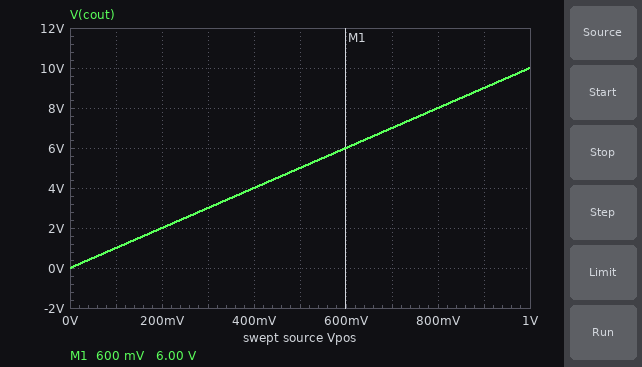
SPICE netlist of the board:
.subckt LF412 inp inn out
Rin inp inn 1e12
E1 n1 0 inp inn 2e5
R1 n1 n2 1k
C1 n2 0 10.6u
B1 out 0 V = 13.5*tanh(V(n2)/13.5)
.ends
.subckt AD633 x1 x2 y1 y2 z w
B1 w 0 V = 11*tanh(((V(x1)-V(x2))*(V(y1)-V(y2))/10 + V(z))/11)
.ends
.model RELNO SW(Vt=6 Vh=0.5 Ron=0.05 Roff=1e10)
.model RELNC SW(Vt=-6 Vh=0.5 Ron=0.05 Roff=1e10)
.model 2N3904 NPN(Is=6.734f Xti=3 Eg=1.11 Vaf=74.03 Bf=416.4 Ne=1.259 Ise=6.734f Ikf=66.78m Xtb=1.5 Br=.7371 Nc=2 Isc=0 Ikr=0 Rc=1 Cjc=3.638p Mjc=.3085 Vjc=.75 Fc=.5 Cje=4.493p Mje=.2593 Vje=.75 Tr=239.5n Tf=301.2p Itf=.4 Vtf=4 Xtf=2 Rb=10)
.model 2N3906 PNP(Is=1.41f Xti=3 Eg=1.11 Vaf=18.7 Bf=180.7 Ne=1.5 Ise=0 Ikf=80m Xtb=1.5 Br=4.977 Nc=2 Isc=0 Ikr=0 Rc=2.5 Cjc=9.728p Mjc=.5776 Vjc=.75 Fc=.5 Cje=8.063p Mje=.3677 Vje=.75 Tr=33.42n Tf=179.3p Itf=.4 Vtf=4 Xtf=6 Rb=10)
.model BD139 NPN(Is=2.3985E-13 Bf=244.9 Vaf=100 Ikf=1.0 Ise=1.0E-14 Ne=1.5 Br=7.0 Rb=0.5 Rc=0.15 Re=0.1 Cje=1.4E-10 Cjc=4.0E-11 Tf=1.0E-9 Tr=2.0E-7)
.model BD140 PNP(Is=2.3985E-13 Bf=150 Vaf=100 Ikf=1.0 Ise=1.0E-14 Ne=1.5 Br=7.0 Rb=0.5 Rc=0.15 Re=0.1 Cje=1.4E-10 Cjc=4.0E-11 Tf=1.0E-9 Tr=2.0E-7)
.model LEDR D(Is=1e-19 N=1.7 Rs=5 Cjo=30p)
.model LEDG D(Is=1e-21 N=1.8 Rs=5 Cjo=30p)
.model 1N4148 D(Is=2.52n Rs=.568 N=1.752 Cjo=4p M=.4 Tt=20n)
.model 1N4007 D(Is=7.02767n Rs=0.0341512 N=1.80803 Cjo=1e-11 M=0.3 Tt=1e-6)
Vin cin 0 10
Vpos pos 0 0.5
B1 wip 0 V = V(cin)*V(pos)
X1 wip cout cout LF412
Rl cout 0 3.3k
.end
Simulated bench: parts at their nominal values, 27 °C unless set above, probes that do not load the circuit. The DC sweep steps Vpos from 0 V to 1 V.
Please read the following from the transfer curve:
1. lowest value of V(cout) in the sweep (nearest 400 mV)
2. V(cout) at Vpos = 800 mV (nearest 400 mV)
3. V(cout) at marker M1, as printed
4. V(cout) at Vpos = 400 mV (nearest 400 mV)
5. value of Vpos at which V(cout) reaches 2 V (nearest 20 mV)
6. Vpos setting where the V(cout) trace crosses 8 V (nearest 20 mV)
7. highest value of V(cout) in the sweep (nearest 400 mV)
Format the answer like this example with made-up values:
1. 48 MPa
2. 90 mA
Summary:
1. 0 V
2. 8.0 V
3. 6.00 V
4. 4.0 V
5. 200 mV
6. 800 mV
7. 10.0 V
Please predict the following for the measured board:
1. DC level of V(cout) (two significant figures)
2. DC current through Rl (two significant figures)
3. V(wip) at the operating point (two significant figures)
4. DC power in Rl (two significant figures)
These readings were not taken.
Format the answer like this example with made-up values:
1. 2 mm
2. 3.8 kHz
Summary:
1. 5.0 V
2. 1.5 mA
3. 5.0 V
4. 7.6 mW
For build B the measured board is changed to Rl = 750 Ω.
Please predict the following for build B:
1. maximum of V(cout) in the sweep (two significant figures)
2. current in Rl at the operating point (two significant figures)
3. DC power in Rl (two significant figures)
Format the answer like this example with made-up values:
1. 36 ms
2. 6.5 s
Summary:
1. 10 V
2. 6.7 mA
3. 33 mW
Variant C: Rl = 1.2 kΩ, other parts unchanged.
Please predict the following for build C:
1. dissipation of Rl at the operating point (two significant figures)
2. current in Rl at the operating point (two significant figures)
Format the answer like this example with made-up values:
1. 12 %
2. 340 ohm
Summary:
1. 21 mW
2. 4.2 mA
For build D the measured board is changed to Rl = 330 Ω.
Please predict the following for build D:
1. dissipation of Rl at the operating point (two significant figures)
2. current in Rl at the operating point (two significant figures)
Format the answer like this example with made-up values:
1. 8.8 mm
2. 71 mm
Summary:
1. 76 mW
2. 15 mA
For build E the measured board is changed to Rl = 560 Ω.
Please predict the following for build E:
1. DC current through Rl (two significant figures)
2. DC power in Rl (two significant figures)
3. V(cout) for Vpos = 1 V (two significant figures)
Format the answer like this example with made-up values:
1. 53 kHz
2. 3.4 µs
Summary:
1. 8.9 mA
2. 45 mW
3. 10 V
